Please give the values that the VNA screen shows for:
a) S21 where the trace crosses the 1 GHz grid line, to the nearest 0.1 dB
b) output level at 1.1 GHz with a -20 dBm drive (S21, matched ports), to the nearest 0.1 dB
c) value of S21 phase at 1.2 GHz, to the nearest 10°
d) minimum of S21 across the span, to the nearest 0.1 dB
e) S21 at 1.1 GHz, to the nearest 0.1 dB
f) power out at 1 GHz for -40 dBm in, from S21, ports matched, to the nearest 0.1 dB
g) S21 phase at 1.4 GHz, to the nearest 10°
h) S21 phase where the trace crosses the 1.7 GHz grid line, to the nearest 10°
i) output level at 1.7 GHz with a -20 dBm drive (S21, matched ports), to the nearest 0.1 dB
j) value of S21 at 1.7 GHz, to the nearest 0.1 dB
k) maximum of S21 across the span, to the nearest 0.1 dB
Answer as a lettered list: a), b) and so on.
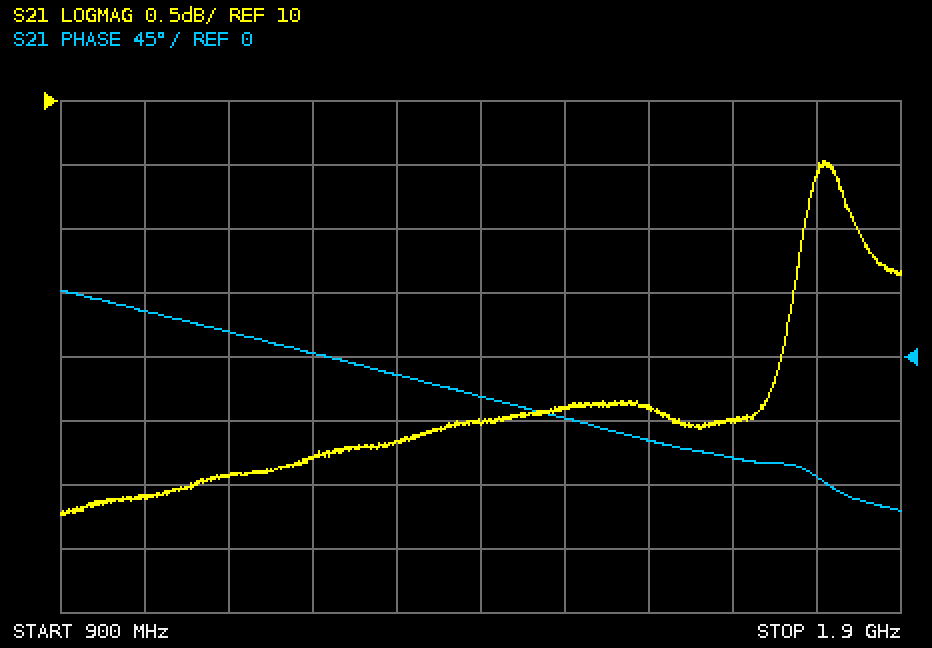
a) 6.9 dB
b) -12.9 dBm
c) 0°
d) 6.8 dB
e) 7.1 dB
f) -33.1 dBm
g) -30°
h) -70°
i) -12.5 dBm
j) 7.5 dB
k) 9.5 dB
